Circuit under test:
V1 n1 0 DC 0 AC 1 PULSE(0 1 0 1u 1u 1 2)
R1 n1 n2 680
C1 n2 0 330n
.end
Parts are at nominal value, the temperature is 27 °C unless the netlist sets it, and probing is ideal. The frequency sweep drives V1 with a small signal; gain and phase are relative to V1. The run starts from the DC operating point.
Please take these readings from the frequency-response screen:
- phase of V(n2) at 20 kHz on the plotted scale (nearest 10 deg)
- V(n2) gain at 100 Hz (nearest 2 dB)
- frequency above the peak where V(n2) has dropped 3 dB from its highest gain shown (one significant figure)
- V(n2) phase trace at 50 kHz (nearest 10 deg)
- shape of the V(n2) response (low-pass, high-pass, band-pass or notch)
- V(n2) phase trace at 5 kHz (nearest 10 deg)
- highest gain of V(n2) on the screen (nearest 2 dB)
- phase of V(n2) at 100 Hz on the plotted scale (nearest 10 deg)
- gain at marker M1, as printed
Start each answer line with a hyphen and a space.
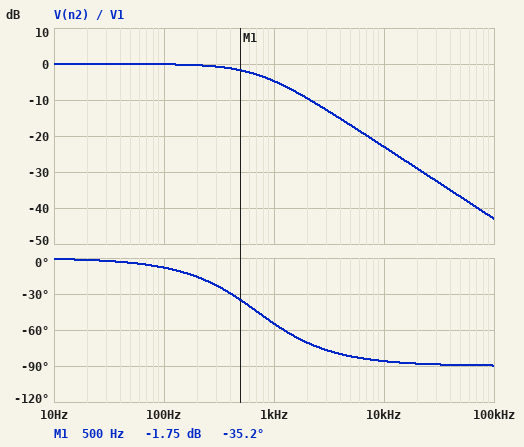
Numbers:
- -90 deg
- 0 dB
- 700 Hz
- -90 deg
- low-pass
- -80 deg
- 0 dB
- -10 deg
- -1.75 dB
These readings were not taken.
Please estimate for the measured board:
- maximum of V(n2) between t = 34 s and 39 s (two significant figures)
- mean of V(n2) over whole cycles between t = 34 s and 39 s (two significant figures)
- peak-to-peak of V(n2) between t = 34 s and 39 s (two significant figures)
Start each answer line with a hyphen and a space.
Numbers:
- 1.0 V
- 500 mV
- 1.0 V
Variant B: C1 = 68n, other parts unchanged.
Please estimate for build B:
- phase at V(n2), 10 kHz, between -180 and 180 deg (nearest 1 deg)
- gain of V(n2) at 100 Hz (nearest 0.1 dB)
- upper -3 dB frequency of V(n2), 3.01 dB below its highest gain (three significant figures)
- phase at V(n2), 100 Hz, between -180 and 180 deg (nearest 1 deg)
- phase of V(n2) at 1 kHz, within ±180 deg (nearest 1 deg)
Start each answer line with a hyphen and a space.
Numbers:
- -71 deg
- 0 dB
- 3.44 kHz
- -2 deg
- -16 deg
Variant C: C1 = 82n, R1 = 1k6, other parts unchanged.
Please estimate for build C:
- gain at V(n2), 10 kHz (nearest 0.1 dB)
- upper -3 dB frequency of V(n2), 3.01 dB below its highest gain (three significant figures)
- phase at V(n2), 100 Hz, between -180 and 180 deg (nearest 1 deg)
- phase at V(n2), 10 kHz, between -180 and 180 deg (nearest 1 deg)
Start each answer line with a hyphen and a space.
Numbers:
- -18.4 dB
- 1.21 kHz
- -5 deg
- -83 deg
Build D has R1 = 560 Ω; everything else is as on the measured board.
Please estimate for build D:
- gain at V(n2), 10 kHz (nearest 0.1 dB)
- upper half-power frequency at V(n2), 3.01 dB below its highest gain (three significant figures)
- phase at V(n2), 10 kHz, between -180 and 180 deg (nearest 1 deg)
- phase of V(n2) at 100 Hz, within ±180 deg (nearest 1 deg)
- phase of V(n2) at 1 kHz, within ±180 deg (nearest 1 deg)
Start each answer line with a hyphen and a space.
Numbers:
- -21.3 dB
- 861 Hz
- -85 deg
- -7 deg
- -49 deg
